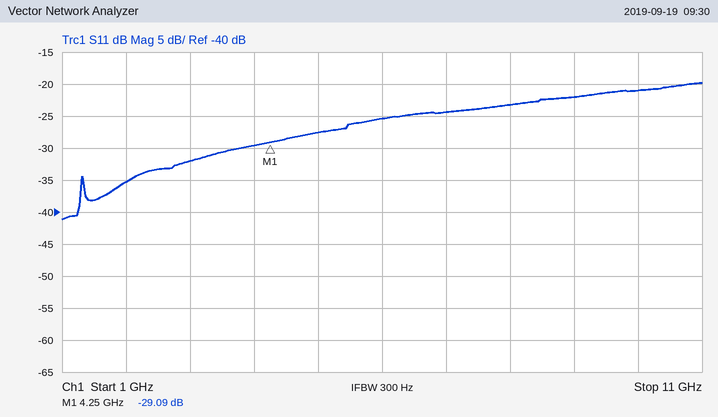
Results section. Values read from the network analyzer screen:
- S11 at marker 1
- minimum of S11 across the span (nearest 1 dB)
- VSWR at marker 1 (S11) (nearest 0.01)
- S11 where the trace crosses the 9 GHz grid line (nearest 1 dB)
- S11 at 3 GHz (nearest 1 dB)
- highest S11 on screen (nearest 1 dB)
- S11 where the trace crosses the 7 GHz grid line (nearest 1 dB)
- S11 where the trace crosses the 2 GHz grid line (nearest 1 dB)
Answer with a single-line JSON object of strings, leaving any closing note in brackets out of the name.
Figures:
{"S11 at marker 1": "-29.09 dB", "minimum of S11 across the span": "-41 dB", "VSWR at marker 1 (S11)": "1.07", "S11 where the trace crosses the 9 GHz grid line": "-22 dB", "S11 at 3 GHz": "-32 dB", "highest S11 on screen": "-20 dB", "S11 where the trace crosses the 7 GHz grid line": "-24 dB", "S11 where the trace crosses the 2 GHz grid line": "-35 dB"}
